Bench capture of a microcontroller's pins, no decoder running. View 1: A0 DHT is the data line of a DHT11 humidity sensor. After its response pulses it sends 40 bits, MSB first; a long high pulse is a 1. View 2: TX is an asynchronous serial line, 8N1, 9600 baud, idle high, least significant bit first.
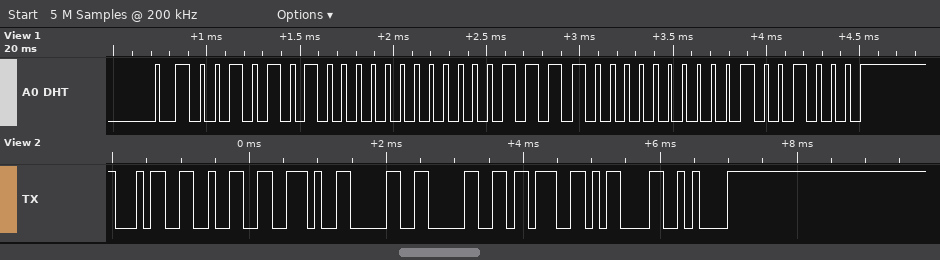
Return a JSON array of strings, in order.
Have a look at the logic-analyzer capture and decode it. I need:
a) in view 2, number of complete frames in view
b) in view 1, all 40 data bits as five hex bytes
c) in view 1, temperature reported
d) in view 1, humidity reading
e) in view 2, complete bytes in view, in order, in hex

["8", "2A 00 1E 00 48", "30.0 °C", "42 %", "0x34 0x32 0x2E 0x30 0x30 0x3B 0x0D 0x0A"]
